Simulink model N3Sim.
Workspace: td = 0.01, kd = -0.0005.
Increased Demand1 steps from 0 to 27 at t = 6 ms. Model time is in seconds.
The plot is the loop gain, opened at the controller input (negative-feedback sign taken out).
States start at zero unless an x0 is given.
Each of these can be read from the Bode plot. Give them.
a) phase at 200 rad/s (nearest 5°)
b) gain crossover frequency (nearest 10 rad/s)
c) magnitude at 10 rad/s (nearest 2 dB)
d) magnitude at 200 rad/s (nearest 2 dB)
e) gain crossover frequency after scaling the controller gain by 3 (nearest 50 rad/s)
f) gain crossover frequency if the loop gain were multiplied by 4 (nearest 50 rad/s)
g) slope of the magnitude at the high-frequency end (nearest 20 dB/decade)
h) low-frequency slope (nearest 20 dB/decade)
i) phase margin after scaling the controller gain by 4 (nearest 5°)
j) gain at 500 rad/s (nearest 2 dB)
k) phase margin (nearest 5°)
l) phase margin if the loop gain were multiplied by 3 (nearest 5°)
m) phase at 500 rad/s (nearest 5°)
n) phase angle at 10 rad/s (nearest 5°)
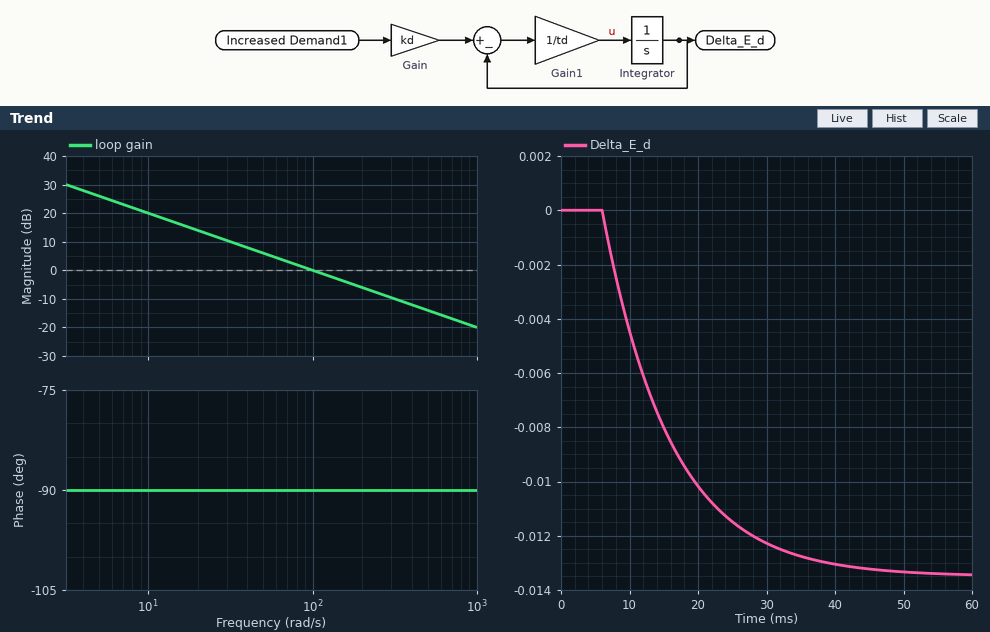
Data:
-90°
100 rad/s
20 dB
-6 dB
300 rad/s
400 rad/s
-20 dB/decade
-20 dB/decade
90°
-14 dB
90°
90°
-90°
-90°
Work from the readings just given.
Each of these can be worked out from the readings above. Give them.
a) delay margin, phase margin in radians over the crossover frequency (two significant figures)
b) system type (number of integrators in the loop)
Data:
0.016 s
1
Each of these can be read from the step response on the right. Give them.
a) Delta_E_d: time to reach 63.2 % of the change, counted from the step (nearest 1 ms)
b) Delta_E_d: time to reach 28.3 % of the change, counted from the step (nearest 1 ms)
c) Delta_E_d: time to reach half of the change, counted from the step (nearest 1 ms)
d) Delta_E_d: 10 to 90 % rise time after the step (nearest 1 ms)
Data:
10 ms
3 ms
7 ms
22 ms
